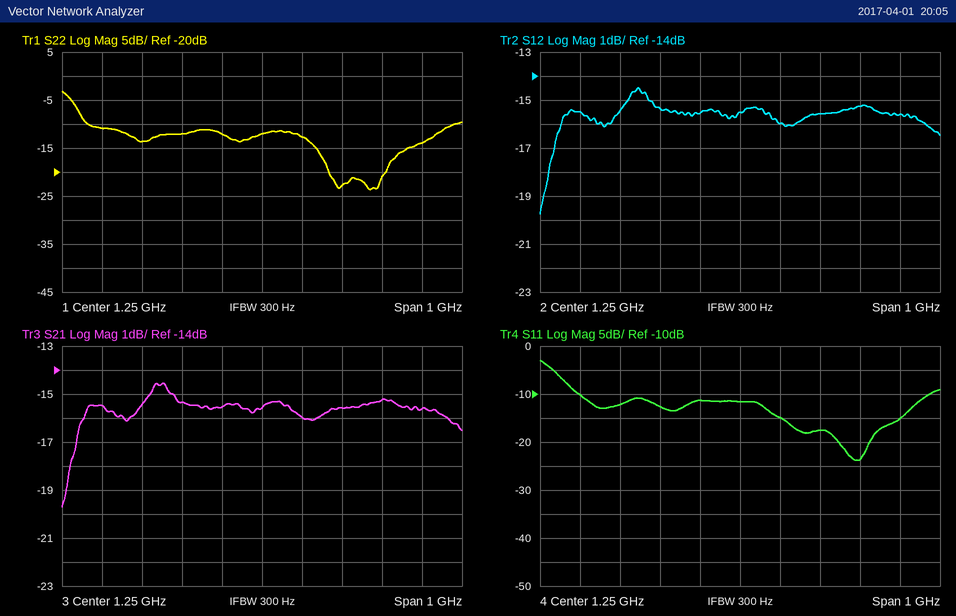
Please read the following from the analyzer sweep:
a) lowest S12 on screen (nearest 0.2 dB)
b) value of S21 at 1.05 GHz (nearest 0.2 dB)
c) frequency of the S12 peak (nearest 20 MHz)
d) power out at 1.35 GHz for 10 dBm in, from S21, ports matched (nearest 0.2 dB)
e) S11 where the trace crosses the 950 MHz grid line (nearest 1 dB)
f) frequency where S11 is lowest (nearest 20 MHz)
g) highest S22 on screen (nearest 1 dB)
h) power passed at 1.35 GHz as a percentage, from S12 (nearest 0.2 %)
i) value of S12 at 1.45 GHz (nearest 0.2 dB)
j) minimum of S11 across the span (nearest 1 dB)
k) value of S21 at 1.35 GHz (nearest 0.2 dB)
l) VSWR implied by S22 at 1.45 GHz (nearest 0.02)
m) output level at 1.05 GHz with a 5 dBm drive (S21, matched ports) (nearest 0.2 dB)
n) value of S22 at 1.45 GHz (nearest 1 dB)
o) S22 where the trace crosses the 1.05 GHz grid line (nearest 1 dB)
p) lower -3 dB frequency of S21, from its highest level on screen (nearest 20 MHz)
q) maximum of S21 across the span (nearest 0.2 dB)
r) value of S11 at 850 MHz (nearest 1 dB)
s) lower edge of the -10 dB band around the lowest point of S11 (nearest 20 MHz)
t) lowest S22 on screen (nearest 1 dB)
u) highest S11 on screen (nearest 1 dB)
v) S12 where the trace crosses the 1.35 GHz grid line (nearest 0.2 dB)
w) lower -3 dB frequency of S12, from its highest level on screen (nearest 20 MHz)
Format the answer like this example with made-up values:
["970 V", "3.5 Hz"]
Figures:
["-19.8 dB", "-15.4 dB", "1.00 GHz", "-6.0 dBm", "-12 dB", "1.54 GHz", "-3 dB", "2.6 %", "-15.6 dB", "-24 dB", "-16.0 dB", "1.16", "-10.4 dBm", "-23 dB", "-12 dB", "780 MHz", "-14.6 dB", "-10 dB", "840 MHz", "-24 dB", "-3 dB", "-16.0 dB", "780 MHz"]
